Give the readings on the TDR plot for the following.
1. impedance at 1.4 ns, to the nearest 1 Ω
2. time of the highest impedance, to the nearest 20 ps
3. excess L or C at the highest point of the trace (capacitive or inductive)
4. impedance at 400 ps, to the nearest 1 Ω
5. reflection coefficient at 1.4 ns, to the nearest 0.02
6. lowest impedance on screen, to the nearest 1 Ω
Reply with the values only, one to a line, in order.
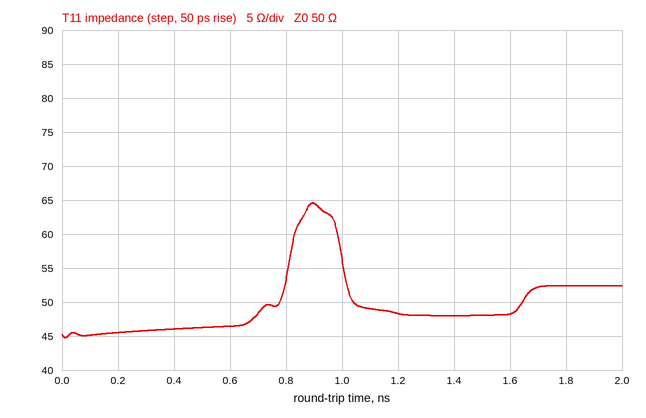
48 Ω
900 ps
inductive
46 Ω
-0.02
45 Ω
